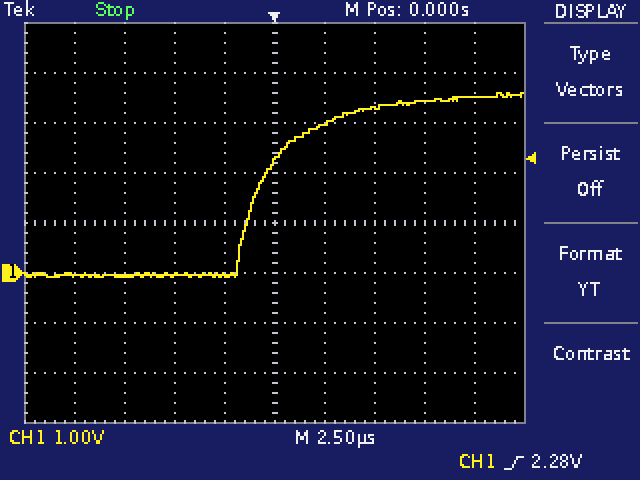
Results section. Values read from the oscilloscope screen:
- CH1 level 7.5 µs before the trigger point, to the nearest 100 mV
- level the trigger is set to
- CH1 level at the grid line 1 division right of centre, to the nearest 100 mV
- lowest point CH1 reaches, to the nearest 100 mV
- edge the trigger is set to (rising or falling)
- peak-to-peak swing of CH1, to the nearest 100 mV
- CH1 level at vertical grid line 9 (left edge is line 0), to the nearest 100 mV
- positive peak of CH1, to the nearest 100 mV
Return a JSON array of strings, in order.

["-100 mV", "2.28 V", "3.0 V", "-100 mV", "rising", "3.7 V", "3.5 V", "3.6 V"]
